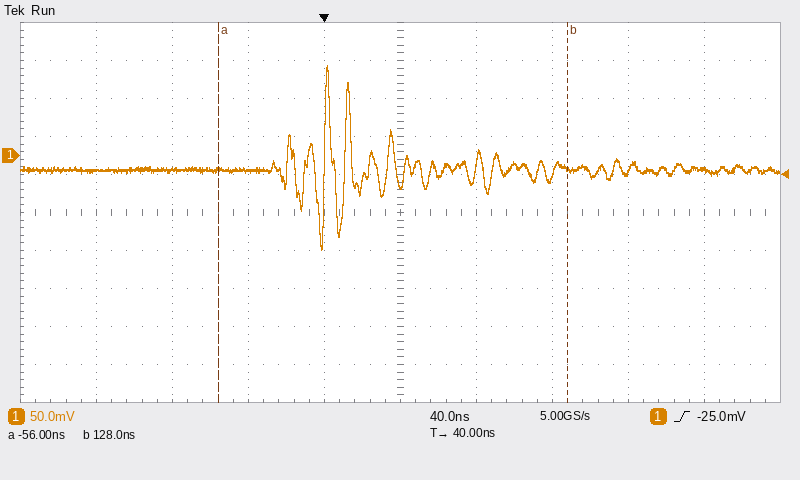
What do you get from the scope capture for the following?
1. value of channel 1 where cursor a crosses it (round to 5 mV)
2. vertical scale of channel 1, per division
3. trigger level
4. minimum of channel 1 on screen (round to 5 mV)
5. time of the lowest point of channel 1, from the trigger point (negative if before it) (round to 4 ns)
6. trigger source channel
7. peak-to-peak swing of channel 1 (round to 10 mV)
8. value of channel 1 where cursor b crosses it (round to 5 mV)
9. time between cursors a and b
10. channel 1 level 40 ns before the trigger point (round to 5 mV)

-20 mV
50 mV
-25.0 mV
-125 mV
0 ns
channel 1
240 mV
-15 mV
184 ns
-20 mV
